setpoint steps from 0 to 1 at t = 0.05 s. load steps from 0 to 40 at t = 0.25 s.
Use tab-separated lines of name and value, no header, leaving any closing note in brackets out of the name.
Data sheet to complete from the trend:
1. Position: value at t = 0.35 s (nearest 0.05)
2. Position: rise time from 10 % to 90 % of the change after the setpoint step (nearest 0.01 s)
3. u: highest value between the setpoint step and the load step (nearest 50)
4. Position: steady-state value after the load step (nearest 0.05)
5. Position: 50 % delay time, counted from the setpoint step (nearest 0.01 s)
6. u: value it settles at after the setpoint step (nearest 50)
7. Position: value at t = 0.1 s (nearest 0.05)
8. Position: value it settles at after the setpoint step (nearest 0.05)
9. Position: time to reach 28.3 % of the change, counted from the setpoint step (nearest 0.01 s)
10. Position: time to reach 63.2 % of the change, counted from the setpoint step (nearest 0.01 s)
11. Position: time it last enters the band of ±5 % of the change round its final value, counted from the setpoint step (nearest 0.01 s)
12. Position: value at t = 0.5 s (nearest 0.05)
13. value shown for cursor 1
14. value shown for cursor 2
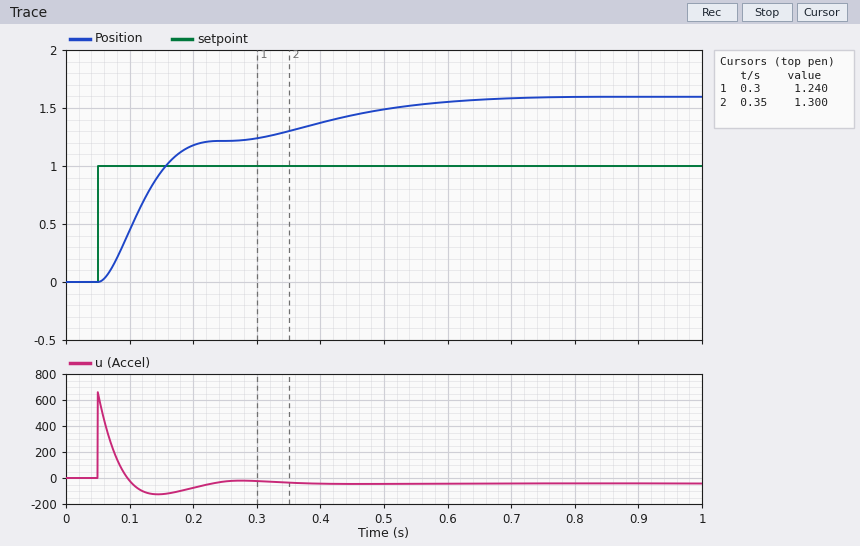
Position: value at t = 0.35 s	1.30
Position: rise time from 10 % to 90 % of the change after the setpoint step	0.10 s
u: highest value between the setpoint step and the load step	650
Position: steady-state value after the load step	1.60
Position: 50 % delay time, counted from the setpoint step	0.06 s
u: value it settles at after the setpoint step	-50
Position: value at t = 0.1 s	0.45
Position: value it settles at after the setpoint step	1.20
Position: time to reach 28.3 % of the change, counted from the setpoint step	0.04 s
Position: time to reach 63.2 % of the change, counted from the setpoint step	0.08 s
Position: time it last enters the band of ±5 % of the change round its final value, counted from the setpoint step	0.14 s
Position: value at t = 0.5 s	1.50
value shown for cursor 1	1.240
value shown for cursor 2	1.300
